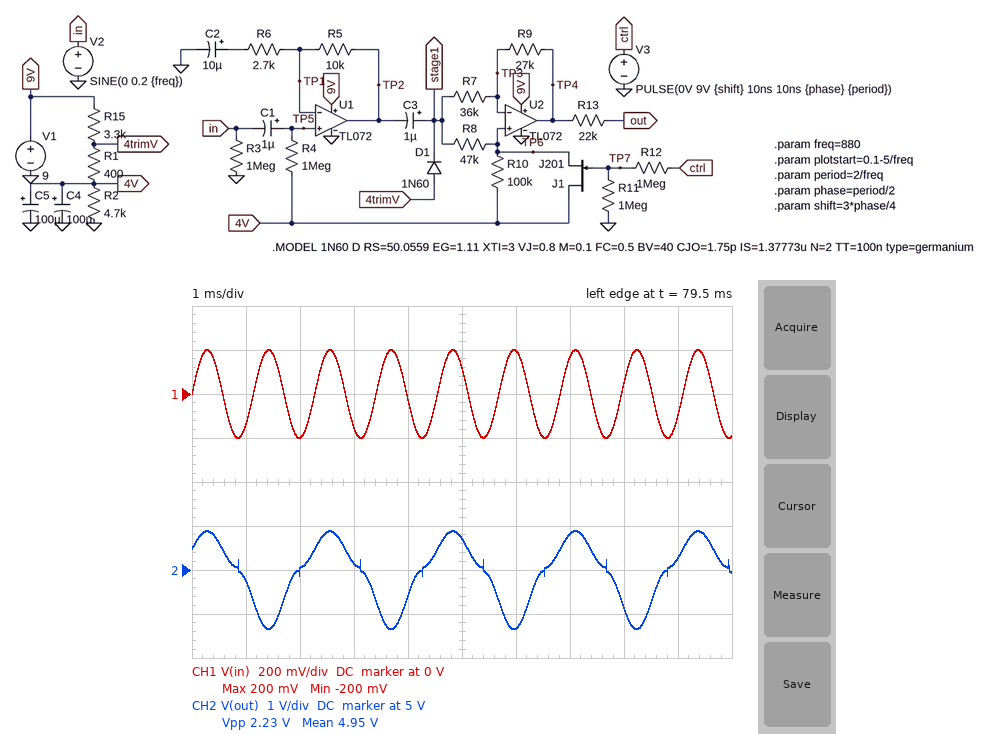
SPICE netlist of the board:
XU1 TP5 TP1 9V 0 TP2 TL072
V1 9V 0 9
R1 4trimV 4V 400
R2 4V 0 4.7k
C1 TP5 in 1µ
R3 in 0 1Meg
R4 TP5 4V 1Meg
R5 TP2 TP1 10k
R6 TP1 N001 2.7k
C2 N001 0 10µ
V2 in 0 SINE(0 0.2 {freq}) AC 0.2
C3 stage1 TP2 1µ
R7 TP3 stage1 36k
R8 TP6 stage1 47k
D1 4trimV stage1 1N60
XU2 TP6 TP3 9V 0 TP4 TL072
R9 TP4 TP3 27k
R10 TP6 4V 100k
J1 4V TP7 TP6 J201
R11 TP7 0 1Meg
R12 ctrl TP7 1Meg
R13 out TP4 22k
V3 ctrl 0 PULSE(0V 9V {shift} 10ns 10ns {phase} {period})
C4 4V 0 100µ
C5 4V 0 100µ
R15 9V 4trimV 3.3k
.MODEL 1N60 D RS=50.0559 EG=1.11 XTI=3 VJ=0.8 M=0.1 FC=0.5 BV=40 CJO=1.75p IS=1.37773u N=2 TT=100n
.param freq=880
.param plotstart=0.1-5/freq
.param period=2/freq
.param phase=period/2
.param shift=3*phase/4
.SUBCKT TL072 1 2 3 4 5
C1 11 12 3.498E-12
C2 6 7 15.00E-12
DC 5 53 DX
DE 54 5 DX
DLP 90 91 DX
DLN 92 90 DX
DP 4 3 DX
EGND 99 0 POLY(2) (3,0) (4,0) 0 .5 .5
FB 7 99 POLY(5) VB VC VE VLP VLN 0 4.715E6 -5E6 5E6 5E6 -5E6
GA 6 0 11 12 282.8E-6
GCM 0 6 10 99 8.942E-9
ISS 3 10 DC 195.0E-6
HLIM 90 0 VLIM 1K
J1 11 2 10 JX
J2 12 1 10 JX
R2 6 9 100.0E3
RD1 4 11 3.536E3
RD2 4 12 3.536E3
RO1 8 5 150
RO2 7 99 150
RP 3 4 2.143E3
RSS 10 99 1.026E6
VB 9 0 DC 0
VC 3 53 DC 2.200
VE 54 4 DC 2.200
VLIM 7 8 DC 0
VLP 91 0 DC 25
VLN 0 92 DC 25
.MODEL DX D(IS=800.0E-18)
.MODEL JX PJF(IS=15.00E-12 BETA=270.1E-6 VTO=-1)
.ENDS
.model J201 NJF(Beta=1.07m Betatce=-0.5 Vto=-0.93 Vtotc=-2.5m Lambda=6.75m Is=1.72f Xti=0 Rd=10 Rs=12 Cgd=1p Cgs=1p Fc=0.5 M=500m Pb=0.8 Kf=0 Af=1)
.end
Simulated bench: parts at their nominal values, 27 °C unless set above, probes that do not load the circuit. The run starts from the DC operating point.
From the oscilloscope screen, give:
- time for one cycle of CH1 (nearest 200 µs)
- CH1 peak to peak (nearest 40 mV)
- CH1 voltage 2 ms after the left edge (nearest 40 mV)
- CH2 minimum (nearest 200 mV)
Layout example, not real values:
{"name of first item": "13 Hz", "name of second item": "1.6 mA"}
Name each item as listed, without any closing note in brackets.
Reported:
{"time for one cycle of CH1": "1.2 ms", "CH1 peak to peak": "400 mV", "CH1 voltage 2 ms after the left edge": "-200 mV", "CH2 minimum": "3.6 V"}
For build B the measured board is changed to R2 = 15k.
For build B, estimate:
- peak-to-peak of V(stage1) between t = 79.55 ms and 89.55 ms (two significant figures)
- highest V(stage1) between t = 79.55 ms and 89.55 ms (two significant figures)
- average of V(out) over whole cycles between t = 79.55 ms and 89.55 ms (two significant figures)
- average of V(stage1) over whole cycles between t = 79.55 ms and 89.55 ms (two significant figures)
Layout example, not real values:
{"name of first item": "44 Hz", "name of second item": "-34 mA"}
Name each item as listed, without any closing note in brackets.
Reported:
{"peak-to-peak of V(stage1) between t = 79.55 ms and 89.55 ms": "960 mV", "highest V(stage1) between t = 79.55 ms and 89.55 ms": "8.1 V", "average of V(out) over whole cycles between t = 79.55 ms and 89.55 ms": "7.4 V", "average of V(stage1) over whole cycles between t = 79.55 ms and 89.55 ms": "7.8 V"}
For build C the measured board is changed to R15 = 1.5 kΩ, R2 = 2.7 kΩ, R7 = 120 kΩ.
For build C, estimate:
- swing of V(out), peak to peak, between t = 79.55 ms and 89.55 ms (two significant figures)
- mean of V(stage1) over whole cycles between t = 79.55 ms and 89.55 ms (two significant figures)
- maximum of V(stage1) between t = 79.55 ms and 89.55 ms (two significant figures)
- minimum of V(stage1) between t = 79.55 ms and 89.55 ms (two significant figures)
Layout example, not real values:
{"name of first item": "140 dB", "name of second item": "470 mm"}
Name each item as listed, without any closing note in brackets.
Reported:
{"swing of V(out), peak to peak, between t = 79.55 ms and 89.55 ms": "1.6 V", "mean of V(stage1) over whole cycles between t = 79.55 ms and 89.55 ms": "6.7 V", "maximum of V(stage1) between t = 79.55 ms and 89.55 ms": "7.6 V", "minimum of V(stage1) between t = 79.55 ms and 89.55 ms": "5.7 V"}
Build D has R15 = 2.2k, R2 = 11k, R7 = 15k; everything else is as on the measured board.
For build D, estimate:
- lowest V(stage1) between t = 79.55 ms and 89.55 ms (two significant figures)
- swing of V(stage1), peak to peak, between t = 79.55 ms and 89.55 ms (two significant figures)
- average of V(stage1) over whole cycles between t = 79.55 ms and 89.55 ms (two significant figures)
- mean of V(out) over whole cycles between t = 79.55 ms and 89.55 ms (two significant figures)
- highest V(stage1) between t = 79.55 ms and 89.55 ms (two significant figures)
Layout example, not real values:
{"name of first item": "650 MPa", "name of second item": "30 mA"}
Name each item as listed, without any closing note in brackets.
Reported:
{"lowest V(stage1) between t = 79.55 ms and 89.55 ms": "7.2 V", "swing of V(stage1), peak to peak, between t = 79.55 ms and 89.55 ms": "880 mV", "average of V(stage1) over whole cycles between t = 79.55 ms and 89.55 ms": "7.8 V", "mean of V(out) over whole cycles between t = 79.55 ms and 89.55 ms": "7.3 V", "highest V(stage1) between t = 79.55 ms and 89.55 ms": "8.1 V"}
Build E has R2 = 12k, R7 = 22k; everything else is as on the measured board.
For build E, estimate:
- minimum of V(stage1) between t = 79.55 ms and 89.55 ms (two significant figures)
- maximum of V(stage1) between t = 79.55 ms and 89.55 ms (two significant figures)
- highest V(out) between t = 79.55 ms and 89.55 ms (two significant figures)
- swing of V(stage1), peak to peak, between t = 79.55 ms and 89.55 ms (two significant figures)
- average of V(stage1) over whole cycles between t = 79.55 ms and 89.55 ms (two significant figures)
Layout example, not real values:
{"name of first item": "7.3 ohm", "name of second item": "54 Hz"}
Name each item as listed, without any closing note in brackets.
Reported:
{"minimum of V(stage1) between t = 79.55 ms and 89.55 ms": "6.8 V", "maximum of V(stage1) between t = 79.55 ms and 89.55 ms": "8.2 V", "highest V(out) between t = 79.55 ms and 89.55 ms": "7.3 V", "swing of V(stage1), peak to peak, between t = 79.55 ms and 89.55 ms": "1.4 V", "average of V(stage1) over whole cycles between t = 79.55 ms and 89.55 ms": "7.6 V"}
